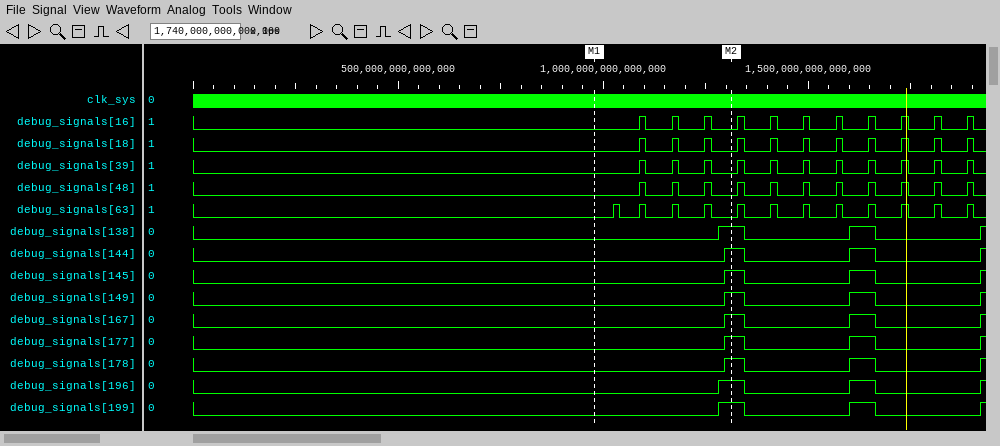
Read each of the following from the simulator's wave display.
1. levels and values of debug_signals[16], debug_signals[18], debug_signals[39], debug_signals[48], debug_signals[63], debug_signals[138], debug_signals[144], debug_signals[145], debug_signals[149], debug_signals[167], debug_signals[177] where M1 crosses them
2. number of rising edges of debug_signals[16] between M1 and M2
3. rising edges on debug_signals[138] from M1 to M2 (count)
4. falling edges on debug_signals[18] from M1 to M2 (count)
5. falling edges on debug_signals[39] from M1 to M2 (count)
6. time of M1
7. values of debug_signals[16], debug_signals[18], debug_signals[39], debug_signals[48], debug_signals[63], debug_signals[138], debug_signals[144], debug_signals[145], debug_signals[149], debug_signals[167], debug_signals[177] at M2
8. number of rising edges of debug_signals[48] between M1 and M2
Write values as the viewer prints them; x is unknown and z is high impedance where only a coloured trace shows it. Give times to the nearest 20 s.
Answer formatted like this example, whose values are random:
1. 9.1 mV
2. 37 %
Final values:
1. debug_signals[16]=0, debug_signals[18]=0, debug_signals[39]=0, debug_signals[48]=0, debug_signals[63]=0, debug_signals[138]=0, debug_signals[144]=0, debug_signals[145]=0, debug_signals[149]=0, debug_signals[167]=0, debug_signals[177]=0
2. 3
3. 1
4. 3
5. 3
6. 980 s
7. debug_signals[16]=0, debug_signals[18]=0, debug_signals[39]=0, debug_signals[48]=0, debug_signals[63]=0, debug_signals[138]=1, debug_signals[144]=1, debug_signals[145]=1, debug_signals[149]=1, debug_signals[167]=1, debug_signals[177]=1
8. 3
